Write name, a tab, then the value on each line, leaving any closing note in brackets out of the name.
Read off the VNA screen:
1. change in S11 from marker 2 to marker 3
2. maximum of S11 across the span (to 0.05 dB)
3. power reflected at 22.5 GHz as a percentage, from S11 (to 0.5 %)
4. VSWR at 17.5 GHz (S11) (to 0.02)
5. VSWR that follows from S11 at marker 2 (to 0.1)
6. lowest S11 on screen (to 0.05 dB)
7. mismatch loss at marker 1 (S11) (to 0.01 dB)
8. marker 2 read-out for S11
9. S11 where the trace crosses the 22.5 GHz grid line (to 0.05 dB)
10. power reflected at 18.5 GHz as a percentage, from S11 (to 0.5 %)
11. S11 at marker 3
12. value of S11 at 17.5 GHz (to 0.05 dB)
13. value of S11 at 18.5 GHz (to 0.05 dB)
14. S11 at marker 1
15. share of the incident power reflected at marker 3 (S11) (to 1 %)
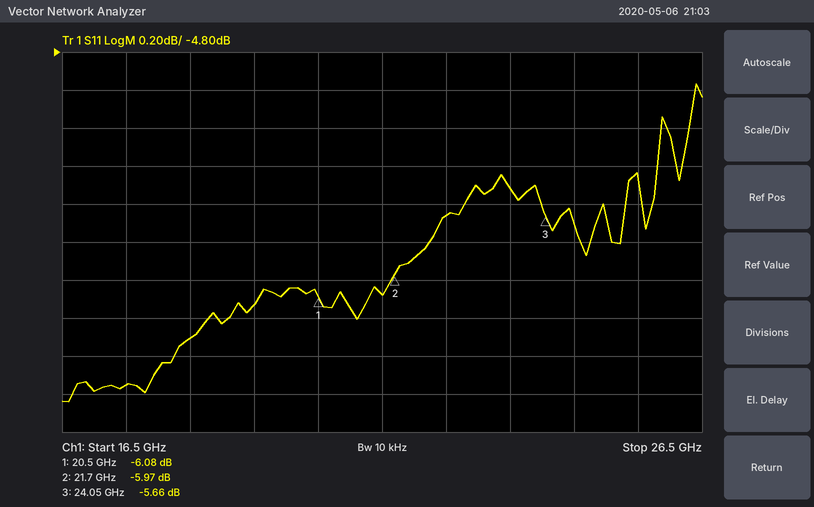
change in S11 from marker 2 to marker 3	0.31 dB
maximum of S11 across the span	-4.95 dB
power reflected at 22.5 GHz as a percentage, from S11	27.0 %
VSWR at 17.5 GHz (S11)	2.78
VSWR that follows from S11 at marker 2	3.0
lowest S11 on screen	-6.65 dB
mismatch loss at marker 1 (S11)	1.23 dB
marker 2 read-out for S11	-5.97 dB
S11 where the trace crosses the 22.5 GHz grid line	-5.65 dB
power reflected at 18.5 GHz as a percentage, from S11	23.5 %
S11 at marker 3	-5.66 dB
value of S11 at 17.5 GHz	-6.55 dB
value of S11 at 18.5 GHz	-6.30 dB
S11 at marker 1	-6.08 dB
share of the incident power reflected at marker 3 (S11)	27 %
